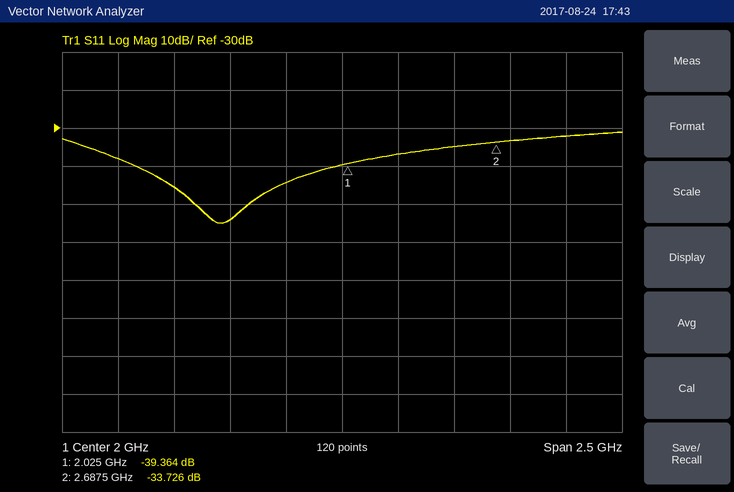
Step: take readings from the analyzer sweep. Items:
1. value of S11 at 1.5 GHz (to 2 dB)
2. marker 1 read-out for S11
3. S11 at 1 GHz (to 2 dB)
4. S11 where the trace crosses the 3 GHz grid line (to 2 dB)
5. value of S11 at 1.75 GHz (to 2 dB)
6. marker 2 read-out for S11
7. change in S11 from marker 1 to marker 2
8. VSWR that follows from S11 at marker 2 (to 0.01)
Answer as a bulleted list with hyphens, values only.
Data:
- -54 dB
- -39.364 dB
- -38 dB
- -32 dB
- -44 dB
- -33.726 dB
- 5.638 dB
- 1.04
